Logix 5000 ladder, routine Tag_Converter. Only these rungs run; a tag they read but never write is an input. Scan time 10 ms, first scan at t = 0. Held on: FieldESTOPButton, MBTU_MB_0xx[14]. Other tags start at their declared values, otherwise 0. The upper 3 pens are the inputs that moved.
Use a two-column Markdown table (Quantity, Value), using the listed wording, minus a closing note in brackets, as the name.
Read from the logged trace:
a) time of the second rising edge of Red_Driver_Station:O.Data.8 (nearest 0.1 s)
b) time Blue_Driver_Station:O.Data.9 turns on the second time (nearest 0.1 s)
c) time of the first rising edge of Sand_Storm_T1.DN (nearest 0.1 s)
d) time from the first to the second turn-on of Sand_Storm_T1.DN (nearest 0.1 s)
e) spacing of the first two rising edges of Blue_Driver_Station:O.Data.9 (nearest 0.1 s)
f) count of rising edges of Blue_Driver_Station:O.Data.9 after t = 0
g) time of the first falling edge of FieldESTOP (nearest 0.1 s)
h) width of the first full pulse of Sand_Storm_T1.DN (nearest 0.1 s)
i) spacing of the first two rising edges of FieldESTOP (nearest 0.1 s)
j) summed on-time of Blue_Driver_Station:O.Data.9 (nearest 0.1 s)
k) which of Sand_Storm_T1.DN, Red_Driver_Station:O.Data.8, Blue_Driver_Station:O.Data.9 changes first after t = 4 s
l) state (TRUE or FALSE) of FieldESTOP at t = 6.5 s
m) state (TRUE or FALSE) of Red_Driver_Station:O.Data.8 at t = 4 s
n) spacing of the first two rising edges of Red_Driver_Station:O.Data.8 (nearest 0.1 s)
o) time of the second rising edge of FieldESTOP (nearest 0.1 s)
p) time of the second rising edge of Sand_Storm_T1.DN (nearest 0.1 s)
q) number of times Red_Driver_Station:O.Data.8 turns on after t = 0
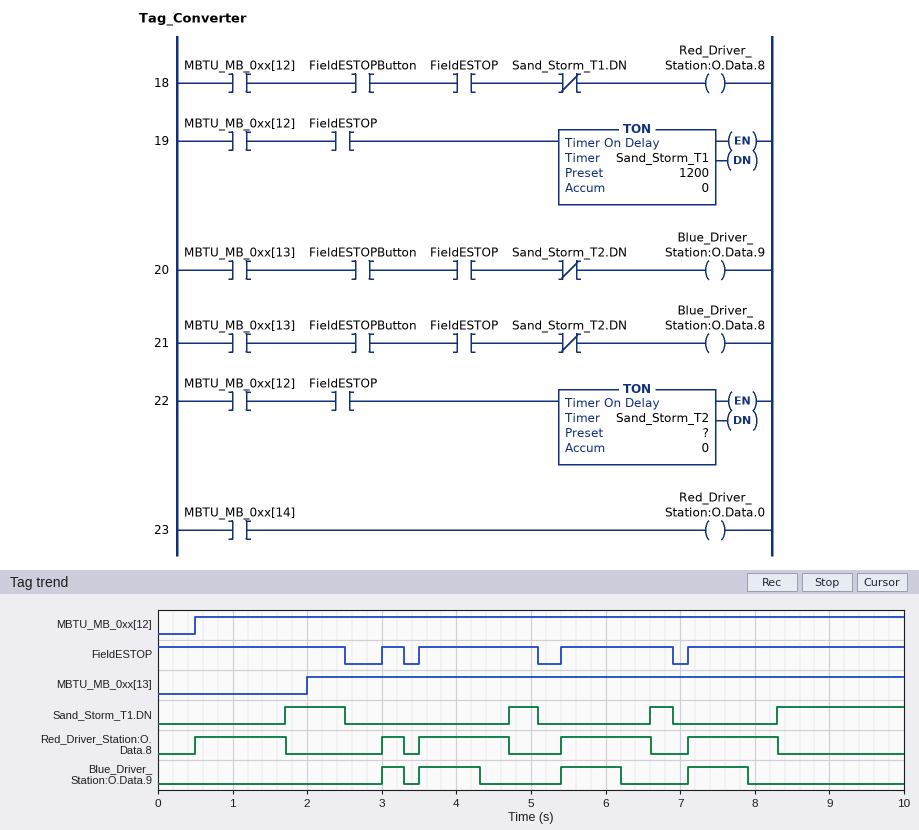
| Quantity | Value |
|---|---|
| time of the second rising edge of Red_Driver_Station:O.Data.8 | 3.0 s |
| time Blue_Driver_Station:O.Data.9 turns on the second time | 3.5 s |
| time of the first rising edge of Sand_Storm_T1.DN | 1.7 s |
| time from the first to the second turn-on of Sand_Storm_T1.DN | 3.0 s |
| spacing of the first two rising edges of Blue_Driver_Station:O.Data.9 | 0.5 s |
| count of rising edges of Blue_Driver_Station:O.Data.9 after t = 0 | 4 |
| time of the first falling edge of FieldESTOP | 2.5 s |
| width of the first full pulse of Sand_Storm_T1.DN | 0.8 s |
| spacing of the first two rising edges of FieldESTOP | 0.5 s |
| summed on-time of Blue_Driver_Station:O.Data.9 | 2.7 s |
| which of Sand_Storm_T1.DN, Red_Driver_Station:O.Data.8, Blue_Driver_Station:O.Data.9 changes first after t = 4 s | Blue_Driver_Station:O.Data.9 |
| state (TRUE or FALSE) of FieldESTOP at t = 6.5 s | TRUE |
| state (TRUE or FALSE) of Red_Driver_Station:O.Data.8 at t = 4 s | TRUE |
| spacing of the first two rising edges of Red_Driver_Station:O.Data.8 | 2.5 s |
| time of the second rising edge of FieldESTOP | 3.5 s |
| time of the second rising edge of Sand_Storm_T1.DN | 4.7 s |
| number of times Red_Driver_Station:O.Data.8 turns on after t = 0 | 5 |
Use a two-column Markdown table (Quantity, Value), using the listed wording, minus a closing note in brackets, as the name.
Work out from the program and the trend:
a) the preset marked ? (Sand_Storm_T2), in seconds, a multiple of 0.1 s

| Quantity | Value |
|---|---|
| the preset marked ? (Sand_Storm_T2), in seconds, a multiple of 0.1 s | 0.8 s |
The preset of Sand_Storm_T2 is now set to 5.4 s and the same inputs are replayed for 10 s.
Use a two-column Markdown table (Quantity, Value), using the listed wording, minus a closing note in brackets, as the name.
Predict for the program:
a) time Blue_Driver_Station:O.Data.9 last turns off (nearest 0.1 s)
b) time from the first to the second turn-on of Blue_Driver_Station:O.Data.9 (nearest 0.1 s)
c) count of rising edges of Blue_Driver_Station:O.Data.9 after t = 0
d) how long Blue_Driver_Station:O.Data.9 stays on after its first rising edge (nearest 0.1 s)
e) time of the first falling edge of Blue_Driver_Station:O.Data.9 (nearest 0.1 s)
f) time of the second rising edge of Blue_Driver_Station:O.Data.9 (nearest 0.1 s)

| Quantity | Value |
|---|---|
| time Blue_Driver_Station:O.Data.9 last turns off | 6.9 s |
| time from the first to the second turn-on of Blue_Driver_Station:O.Data.9 | 1.0 s |
| count of rising edges of Blue_Driver_Station:O.Data.9 after t = 0 | 5 |
| how long Blue_Driver_Station:O.Data.9 stays on after its first rising edge | 0.5 s |
| time of the first falling edge of Blue_Driver_Station:O.Data.9 | 2.5 s |
| time of the second rising edge of Blue_Driver_Station:O.Data.9 | 3.0 s |
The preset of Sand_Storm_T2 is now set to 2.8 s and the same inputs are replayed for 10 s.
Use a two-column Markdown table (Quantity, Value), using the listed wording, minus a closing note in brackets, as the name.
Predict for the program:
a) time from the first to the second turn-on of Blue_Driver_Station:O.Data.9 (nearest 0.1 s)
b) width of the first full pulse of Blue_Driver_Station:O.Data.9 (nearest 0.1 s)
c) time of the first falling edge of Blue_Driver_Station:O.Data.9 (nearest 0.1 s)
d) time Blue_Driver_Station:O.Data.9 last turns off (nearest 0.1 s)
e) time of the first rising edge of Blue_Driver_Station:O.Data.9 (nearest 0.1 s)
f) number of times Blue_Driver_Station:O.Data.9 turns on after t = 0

| Quantity | Value |
|---|---|
| time from the first to the second turn-on of Blue_Driver_Station:O.Data.9 | 1.0 s |
| width of the first full pulse of Blue_Driver_Station:O.Data.9 | 0.5 s |
| time of the first falling edge of Blue_Driver_Station:O.Data.9 | 2.5 s |
| time Blue_Driver_Station:O.Data.9 last turns off | 9.9 s |
| time of the first rising edge of Blue_Driver_Station:O.Data.9 | 2.0 s |
| number of times Blue_Driver_Station:O.Data.9 turns on after t = 0 | 5 |
